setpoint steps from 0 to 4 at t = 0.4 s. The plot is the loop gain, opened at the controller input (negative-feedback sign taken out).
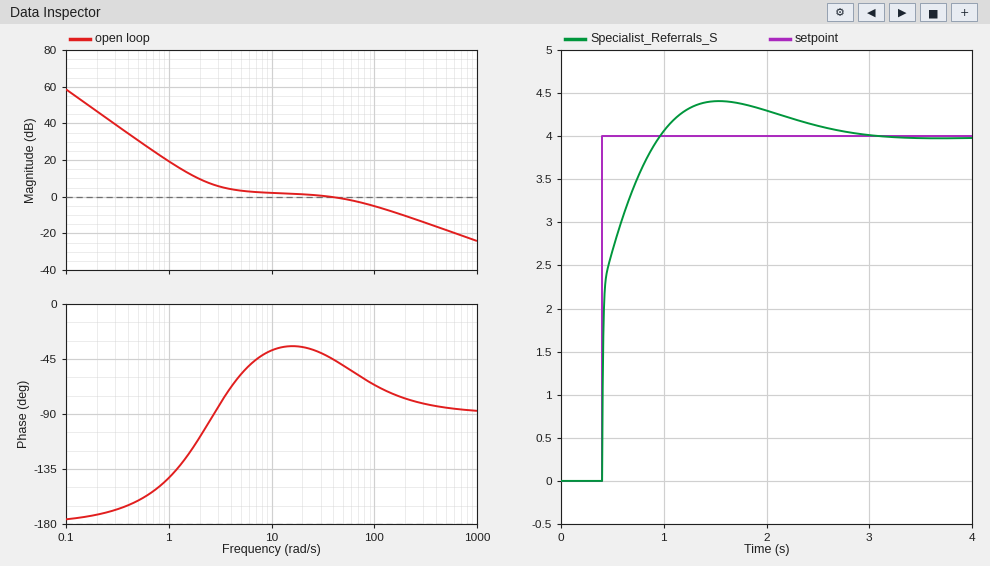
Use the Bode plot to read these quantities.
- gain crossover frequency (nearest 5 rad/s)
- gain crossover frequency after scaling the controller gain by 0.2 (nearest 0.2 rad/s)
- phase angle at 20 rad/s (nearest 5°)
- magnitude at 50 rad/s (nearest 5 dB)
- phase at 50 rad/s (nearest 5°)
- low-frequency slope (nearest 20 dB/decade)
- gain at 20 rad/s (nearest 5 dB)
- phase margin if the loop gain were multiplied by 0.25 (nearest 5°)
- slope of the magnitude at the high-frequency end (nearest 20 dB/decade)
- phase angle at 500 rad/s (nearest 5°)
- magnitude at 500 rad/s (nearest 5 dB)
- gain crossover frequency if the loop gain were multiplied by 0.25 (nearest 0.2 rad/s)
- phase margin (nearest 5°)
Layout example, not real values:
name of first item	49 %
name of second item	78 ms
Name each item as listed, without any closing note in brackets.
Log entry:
gain crossover frequency	35 rad/s
gain crossover frequency after scaling the controller gain by 0.2	1.4 rad/s
phase angle at 20 rad/s	-35°
magnitude at 50 rad/s	0 dB
phase at 50 rad/s	-50°
low-frequency slope	-40 dB/decade
gain at 20 rad/s	0 dB
phase margin if the loop gain were multiplied by 0.25	60°
slope of the magnitude at the high-frequency end	-20 dB/decade
phase angle at 500 rad/s	-85°
magnitude at 500 rad/s	-20 dB
gain crossover frequency if the loop gain were multiplied by 0.25	1.6 rad/s
phase margin	135°
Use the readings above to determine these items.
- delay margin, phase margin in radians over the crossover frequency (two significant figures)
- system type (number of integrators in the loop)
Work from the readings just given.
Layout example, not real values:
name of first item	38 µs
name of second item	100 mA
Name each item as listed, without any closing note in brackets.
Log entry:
delay margin, phase margin in radians over the crossover frequency	0.067 s
system type	2
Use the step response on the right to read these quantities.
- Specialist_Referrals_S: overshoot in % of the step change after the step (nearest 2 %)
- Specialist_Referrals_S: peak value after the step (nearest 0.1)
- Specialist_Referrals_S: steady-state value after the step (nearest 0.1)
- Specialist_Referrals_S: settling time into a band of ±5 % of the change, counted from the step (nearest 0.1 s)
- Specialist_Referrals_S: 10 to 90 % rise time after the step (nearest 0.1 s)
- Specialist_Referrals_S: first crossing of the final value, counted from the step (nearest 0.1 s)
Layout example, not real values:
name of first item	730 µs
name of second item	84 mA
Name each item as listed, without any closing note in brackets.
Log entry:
Specialist_Referrals_S: overshoot in % of the step change after the step	10 %
Specialist_Referrals_S: peak value after the step	4.4
Specialist_Referrals_S: steady-state value after the step	4.0
Specialist_Referrals_S: settling time into a band of ±5 % of the change, counted from the step	1.9 s
Specialist_Referrals_S: 10 to 90 % rise time after the step	0.4 s
Specialist_Referrals_S: first crossing of the final value, counted from the step	0.6 s
